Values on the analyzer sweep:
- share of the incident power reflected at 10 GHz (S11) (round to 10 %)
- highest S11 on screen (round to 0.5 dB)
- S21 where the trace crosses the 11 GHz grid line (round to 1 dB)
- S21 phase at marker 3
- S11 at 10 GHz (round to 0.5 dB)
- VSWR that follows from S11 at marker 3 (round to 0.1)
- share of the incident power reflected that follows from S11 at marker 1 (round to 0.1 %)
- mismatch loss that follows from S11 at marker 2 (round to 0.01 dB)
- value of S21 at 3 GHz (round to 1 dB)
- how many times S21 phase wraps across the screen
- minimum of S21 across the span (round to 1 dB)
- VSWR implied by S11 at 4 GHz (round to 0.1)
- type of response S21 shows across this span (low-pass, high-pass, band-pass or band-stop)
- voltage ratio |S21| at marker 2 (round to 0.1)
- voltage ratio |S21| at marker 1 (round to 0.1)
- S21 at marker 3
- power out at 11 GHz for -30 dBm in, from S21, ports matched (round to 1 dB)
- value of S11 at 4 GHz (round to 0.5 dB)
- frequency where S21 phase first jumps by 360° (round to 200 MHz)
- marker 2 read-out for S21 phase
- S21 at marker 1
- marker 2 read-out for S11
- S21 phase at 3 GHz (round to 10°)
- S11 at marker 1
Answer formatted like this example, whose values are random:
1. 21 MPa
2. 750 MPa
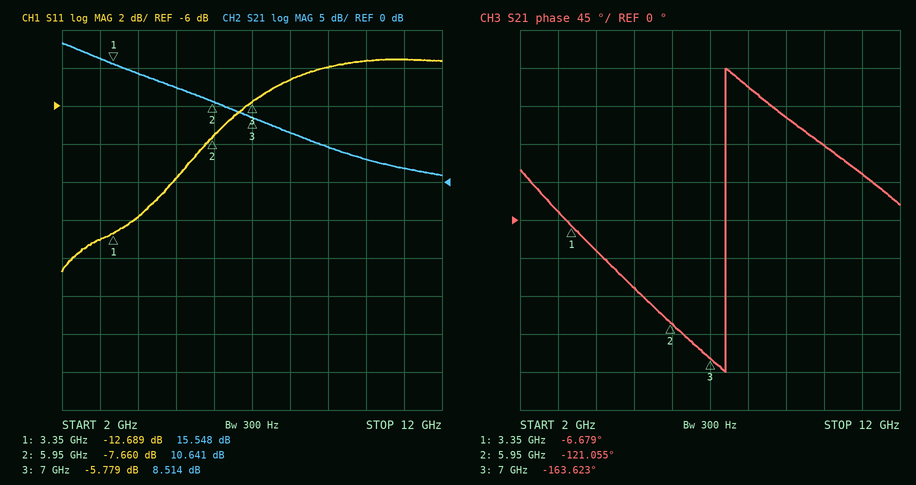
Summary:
1. 40 %
2. -3.5 dB
3. 2 dB
4. -163.623°
5. -3.5 dB
6. 3.1
7. 5.4 %
8. 0.82 dB
9. 16 dB
10. 1
11. 1 dB
12. 1.7
13. low-pass
14. 3.4
15. 6.0
16. 8.514 dB
17. -28 dBm
18. -12.0 dB
19. 7.4 GHz
20. -121.055°
21. 15.548 dB
22. -7.660 dB
23. 10°
24. -12.689 dB
